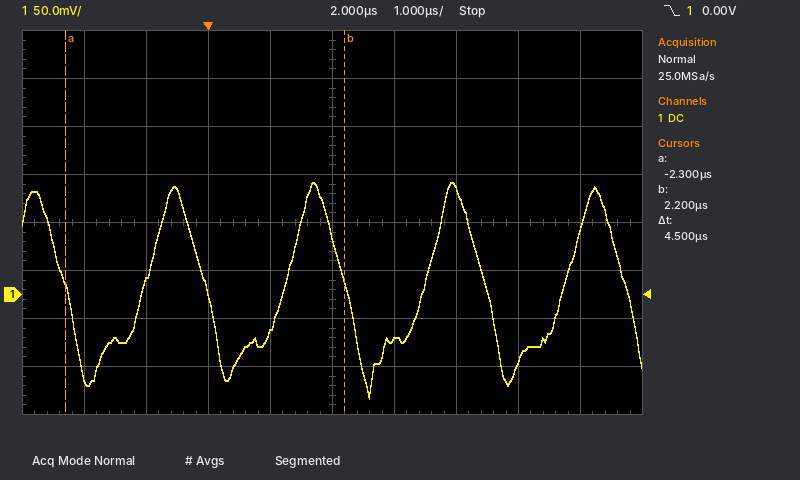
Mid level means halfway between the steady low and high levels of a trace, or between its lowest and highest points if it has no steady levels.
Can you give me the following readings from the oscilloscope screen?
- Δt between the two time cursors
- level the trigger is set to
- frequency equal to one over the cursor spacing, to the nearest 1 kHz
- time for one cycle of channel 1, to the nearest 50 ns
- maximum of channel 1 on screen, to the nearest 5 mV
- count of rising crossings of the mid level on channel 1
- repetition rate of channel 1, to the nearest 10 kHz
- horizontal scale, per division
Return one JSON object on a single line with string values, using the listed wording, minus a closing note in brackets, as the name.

{"Δt between the two time cursors": "4.5 µs", "level the trigger is set to": "0.00 V", "frequency equal to one over the cursor spacing, to the nearest 1 kHz": "222 kHz", "time for one cycle of channel 1, to the nearest 50 ns": "2.25 µs", "maximum of channel 1 on screen, to the nearest 5 mV": "115 mV", "count of rising crossings of the mid level on channel 1": "4", "repetition rate of channel 1, to the nearest 10 kHz": "440 kHz", "horizontal scale, per division": "1 µs"}
